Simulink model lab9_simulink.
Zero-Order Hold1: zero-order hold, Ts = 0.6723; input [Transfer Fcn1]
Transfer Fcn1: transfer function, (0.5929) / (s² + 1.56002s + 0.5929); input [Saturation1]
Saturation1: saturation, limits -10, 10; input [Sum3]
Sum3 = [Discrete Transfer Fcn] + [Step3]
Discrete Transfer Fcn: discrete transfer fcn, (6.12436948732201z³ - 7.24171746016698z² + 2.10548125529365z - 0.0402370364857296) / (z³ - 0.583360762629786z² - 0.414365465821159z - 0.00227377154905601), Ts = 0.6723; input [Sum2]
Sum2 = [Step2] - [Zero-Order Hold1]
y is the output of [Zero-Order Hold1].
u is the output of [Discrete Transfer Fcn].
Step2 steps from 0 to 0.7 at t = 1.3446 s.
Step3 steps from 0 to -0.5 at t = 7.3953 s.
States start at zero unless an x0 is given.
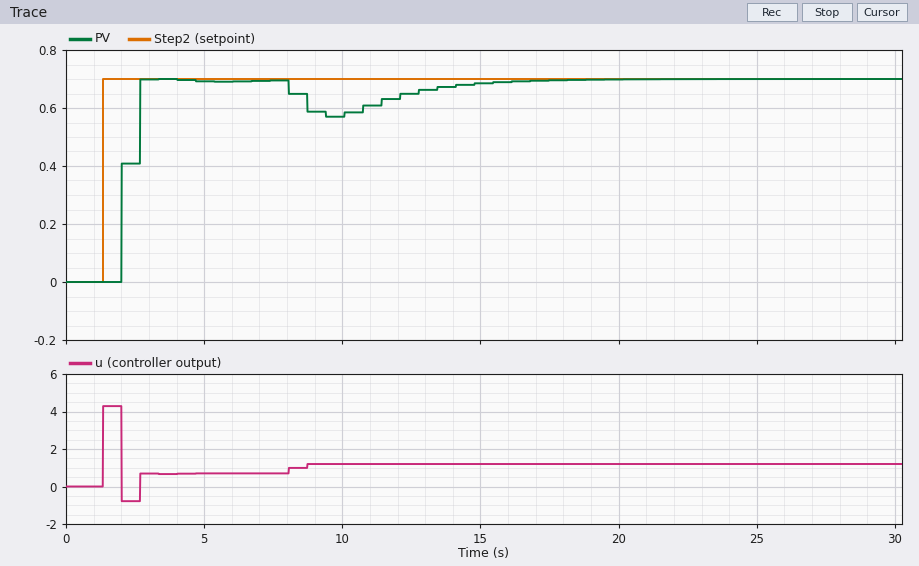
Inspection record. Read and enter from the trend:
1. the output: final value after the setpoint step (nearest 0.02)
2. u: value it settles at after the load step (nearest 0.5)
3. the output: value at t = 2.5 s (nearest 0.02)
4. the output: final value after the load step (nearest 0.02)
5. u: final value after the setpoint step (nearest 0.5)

0.70
1.0
0.40
0.70
0.5
